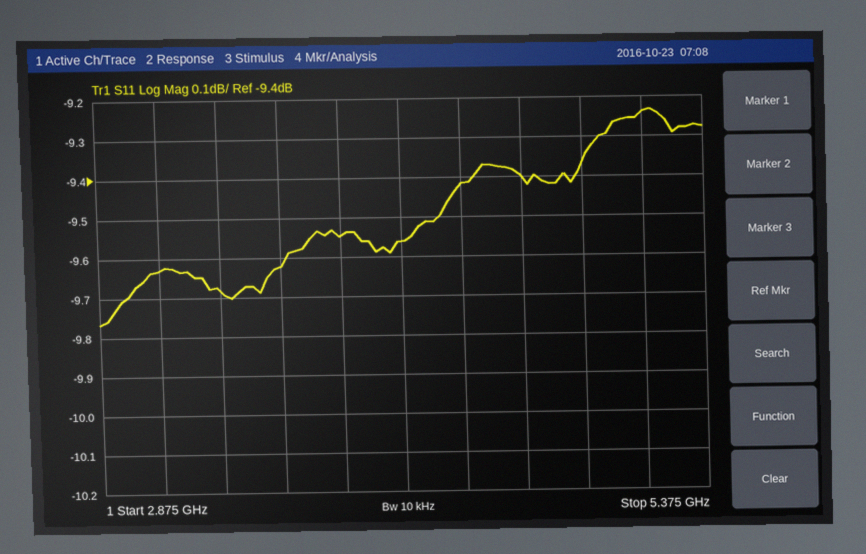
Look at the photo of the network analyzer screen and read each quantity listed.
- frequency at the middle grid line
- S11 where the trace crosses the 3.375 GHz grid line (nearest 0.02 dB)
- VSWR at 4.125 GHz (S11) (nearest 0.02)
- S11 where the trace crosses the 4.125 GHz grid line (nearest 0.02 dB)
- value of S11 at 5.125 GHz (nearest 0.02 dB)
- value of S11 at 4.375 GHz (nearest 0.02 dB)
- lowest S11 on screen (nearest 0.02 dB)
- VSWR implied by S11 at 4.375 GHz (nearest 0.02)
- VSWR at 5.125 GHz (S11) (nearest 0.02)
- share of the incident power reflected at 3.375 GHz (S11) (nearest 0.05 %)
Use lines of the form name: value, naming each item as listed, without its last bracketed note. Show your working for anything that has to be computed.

frequency at the middle grid line: 4.125 GHz
S11 where the trace crosses the 3.375 GHz grid line: -9.68 dB
VSWR at 4.125 GHz (S11): |Γ| = 10^(-9.56/20) = 0.3327; VSWR = (1 + 0.3327)/(1 − 0.3327) ≈ 2.00
S11 where the trace crosses the 4.125 GHz grid line: -9.56 dB
value of S11 at 5.125 GHz: -9.24 dB
value of S11 at 4.375 GHz: -9.42 dB
lowest S11 on screen: -9.76 dB
VSWR implied by S11 at 4.375 GHz: |Γ| = 10^(-9.42/20) = 0.3381; VSWR = (1 + 0.3381)/(1 − 0.3381) ≈ 2.02
VSWR at 5.125 GHz (S11): |Γ| = 10^(-9.24/20) = 0.3451; VSWR = (1 + 0.3451)/(1 − 0.3451) ≈ 2.05, so 2.06 to the nearest 0.02
share of the incident power reflected at 3.375 GHz (S11): 10^(-9.68/10) ≈ 10.8 %, so 10.75 % to the nearest 0.05 %
